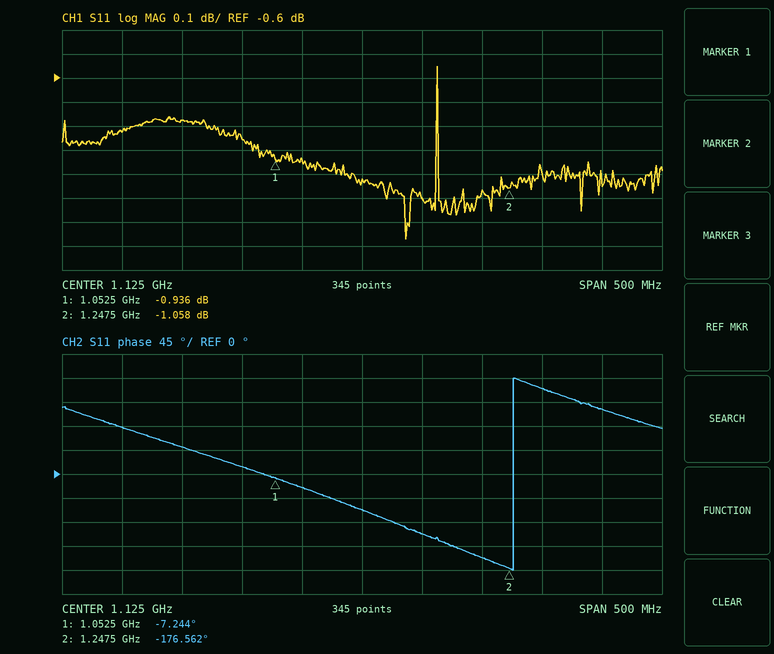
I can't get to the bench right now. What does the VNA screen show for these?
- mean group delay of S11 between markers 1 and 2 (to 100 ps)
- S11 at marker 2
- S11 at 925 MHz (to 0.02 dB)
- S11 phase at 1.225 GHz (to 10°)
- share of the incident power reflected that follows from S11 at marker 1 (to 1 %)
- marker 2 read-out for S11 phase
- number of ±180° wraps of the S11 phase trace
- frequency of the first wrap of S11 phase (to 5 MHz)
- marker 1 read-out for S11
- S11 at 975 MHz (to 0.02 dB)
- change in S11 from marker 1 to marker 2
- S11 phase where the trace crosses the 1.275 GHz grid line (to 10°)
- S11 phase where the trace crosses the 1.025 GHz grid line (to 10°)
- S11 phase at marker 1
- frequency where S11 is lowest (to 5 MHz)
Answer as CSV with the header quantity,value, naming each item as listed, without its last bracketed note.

quantity,value
mean group delay of S11 between markers 1 and 2,2.4 ns
S11 at marker 2,-1.058 dB
S11 at 925 MHz,-0.82 dB
S11 phase at 1.225 GHz,-160°
share of the incident power reflected that follows from S11 at marker 1,81 %
marker 2 read-out for S11 phase,-176.562°
number of ±180° wraps of the S11 phase trace,1
frequency of the first wrap of S11 phase,1.250 GHz
marker 1 read-out for S11,-0.936 dB
S11 at 975 MHz,-0.78 dB
change in S11 from marker 1 to marker 2,-0.122 dB
S11 phase where the trace crosses the 1.275 GHz grid line,160°
S11 phase where the trace crosses the 1.025 GHz grid line,10°
S11 phase at marker 1,-7.244°
frequency where S11 is lowest,1.160 GHz
